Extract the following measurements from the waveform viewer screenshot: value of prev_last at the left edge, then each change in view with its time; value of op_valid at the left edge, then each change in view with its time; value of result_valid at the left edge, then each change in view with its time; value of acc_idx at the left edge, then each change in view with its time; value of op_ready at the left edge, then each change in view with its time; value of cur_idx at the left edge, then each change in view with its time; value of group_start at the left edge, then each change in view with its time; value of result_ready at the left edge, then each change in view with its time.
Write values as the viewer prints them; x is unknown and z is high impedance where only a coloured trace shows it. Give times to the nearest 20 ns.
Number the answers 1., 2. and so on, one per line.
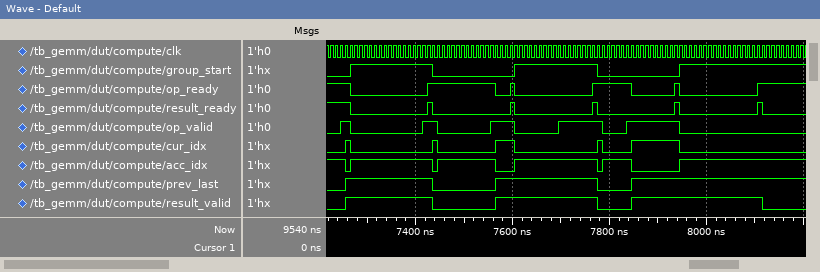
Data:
1. 0, 1 at 7260 ns, 0 at 7440 ns, 1 at 7560 ns, 0 at 7780 ns, 1 at 7840 ns
2. 0, 1 at 7240 ns, 0 at 7260 ns, 1 at 7420 ns, 0 at 7440 ns, 1 at 7560 ns, 0 at 7600 ns, 1 at 7700 ns, 0 at 7780 ns, 1 at 7840 ns, 0 at 7940 ns
3. 0, 1 at 7260 ns, 0 at 7440 ns, 1 at 7560 ns, 0 at 7780 ns, 1 at 7840 ns, 0 at 8120 ns
4. 1, 0 at 7260 ns, 1 at 7260 ns, 0 at 7440 ns, 1 at 7440 ns, 0 at 7560 ns, 1 at 7600 ns, 0 at 7780 ns, 1 at 7780 ns, 0 at 7840 ns, 1 at 7940 ns
5. 1, 0 at 7260 ns, 1 at 7420 ns, 0 at 7560 ns, 1 at 7600 ns, 0 at 7600 ns, 1 at 7760 ns, 0 at 7840 ns, 1 at 7940 ns, 0 at 7940 ns, 1 at 8100 ns
6. 0, 1 at 7260 ns, 0 at 7260 ns, 1 at 7440 ns, 0 at 7440 ns, 1 at 7560 ns, 0 at 7600 ns, 1 at 7780 ns, 0 at 7780 ns, 1 at 7840 ns, 0 at 7940 ns
7. 0, 1 at 7260 ns, 0 at 7440 ns, 1 at 7600 ns, 0 at 7780 ns, 1 at 7940 ns
8. 1, 0 at 7260 ns, 1 at 7420 ns, 0 at 7440 ns, 1 at 7600 ns, 0 at 7600 ns, 1 at 7760 ns, 0 at 7780 ns, 1 at 7940 ns, 0 at 7940 ns, 1 at 8100 ns, 0 at 8120 ns
